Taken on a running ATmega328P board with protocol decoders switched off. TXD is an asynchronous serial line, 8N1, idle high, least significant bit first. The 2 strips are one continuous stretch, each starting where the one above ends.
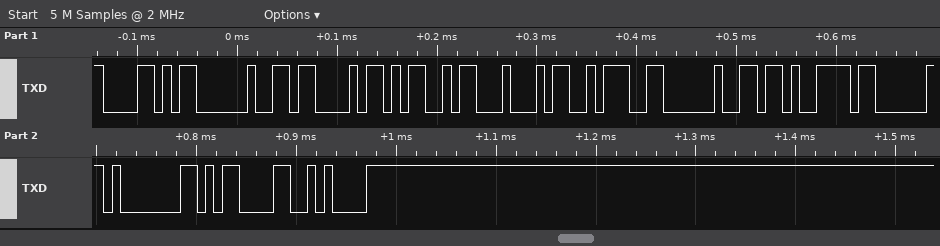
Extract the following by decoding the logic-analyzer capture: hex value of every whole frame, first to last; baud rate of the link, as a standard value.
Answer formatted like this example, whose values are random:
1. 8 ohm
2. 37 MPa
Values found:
1. 0x58 0x20 0x43 0x4D 0x44 0x3A 0x20 0xCB 0x03 0x01 0x0D 0x0A
2. 115200 baud
